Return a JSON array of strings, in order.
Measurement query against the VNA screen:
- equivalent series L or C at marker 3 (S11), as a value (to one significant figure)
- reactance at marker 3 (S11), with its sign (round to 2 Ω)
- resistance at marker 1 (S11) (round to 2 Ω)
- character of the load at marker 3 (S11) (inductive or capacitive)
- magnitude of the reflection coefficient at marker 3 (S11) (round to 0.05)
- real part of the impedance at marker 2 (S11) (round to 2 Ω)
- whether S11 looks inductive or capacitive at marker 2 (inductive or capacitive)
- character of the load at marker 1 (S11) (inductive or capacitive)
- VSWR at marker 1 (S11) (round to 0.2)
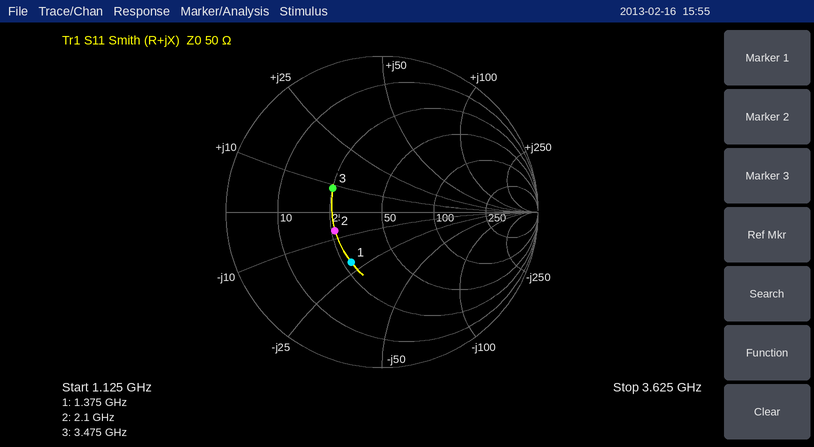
["400 pH", "+8 Ω", "28 Ω", "inductive", "0.35", "26 Ω", "capacitive", "capacitive", "2.2"]
